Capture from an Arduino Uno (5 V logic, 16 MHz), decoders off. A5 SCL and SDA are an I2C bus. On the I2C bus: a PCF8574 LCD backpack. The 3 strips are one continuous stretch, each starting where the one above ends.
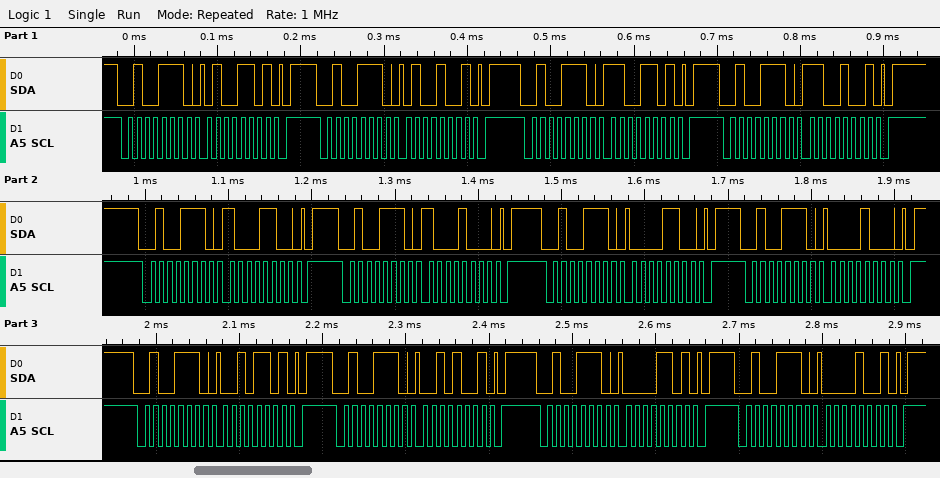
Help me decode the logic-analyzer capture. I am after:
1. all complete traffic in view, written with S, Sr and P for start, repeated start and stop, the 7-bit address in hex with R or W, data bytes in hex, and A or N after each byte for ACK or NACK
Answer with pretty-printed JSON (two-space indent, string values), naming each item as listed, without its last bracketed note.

{
  "all complete traffic in view, written with S, Sr and P for start, repeated start and stop, the 7-bit address in hex with R or W, data bytes in hex, and A or N after each byte for ACK or NACK": "S 27W A 4D A P S 27W A 49 A P S 27W A CD A P S 27W A C9 A P S 27W A 8C A P S 27W A 88 A P S 27W A 0C A P S 27W A 08 A P S 27W A 2D A P S 27W A 29 A P S 27W A 0D A P S 27W A 09 A P"
}
